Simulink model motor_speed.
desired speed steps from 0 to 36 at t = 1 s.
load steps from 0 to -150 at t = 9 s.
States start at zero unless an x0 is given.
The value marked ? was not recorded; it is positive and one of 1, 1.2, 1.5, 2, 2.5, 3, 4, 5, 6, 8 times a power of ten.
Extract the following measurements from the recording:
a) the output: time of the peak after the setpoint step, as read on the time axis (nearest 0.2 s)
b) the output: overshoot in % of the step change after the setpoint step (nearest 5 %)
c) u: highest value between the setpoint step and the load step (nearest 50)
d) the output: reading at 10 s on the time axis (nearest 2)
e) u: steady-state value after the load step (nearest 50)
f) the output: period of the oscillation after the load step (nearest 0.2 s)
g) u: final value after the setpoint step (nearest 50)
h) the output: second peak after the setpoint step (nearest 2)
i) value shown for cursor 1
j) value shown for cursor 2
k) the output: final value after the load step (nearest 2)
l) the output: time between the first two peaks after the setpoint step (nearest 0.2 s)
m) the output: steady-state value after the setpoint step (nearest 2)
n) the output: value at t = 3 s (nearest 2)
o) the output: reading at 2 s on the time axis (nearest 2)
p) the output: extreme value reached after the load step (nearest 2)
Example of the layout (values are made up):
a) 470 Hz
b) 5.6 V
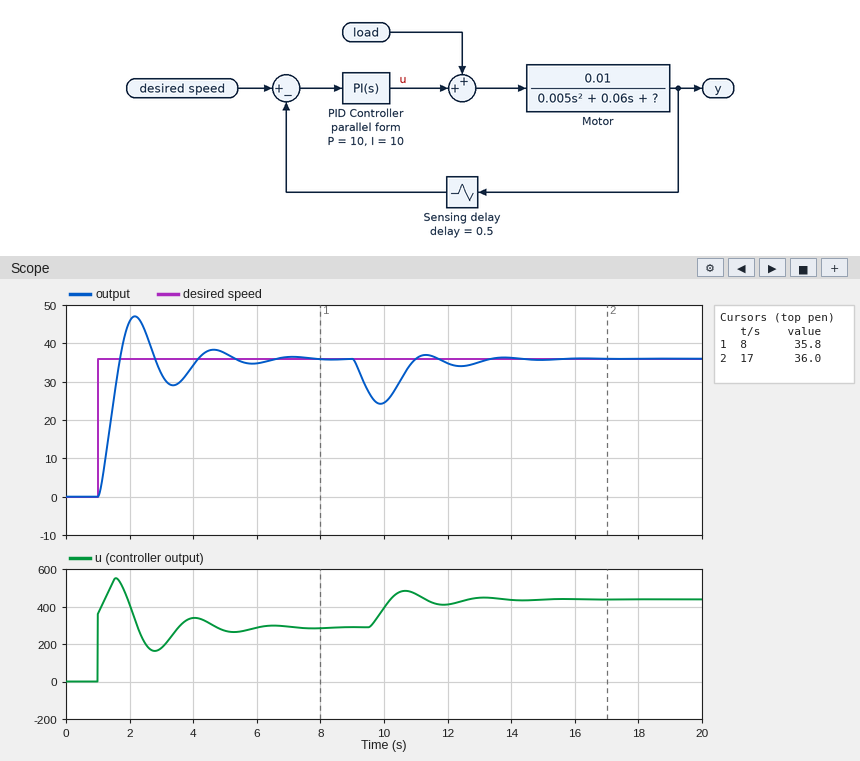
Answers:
a) 2.2 s
b) 30 %
c) 550
d) 24
e) 450
f) 2.6 s
g) 300
h) 38
i) 35.8
j) 36.0
k) 36
l) 2.4 s
m) 36
n) 32
o) 46
p) 24
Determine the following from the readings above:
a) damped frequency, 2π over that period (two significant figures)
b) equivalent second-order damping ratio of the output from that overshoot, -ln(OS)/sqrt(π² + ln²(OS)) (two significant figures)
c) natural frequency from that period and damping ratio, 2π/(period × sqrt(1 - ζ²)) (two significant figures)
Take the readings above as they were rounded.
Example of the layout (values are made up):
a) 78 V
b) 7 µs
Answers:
a) 2.6 rad/s
b) 0.36
c) 2.8 rad/s
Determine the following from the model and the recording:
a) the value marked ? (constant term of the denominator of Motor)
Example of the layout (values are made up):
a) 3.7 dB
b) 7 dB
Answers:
a) 0.08
